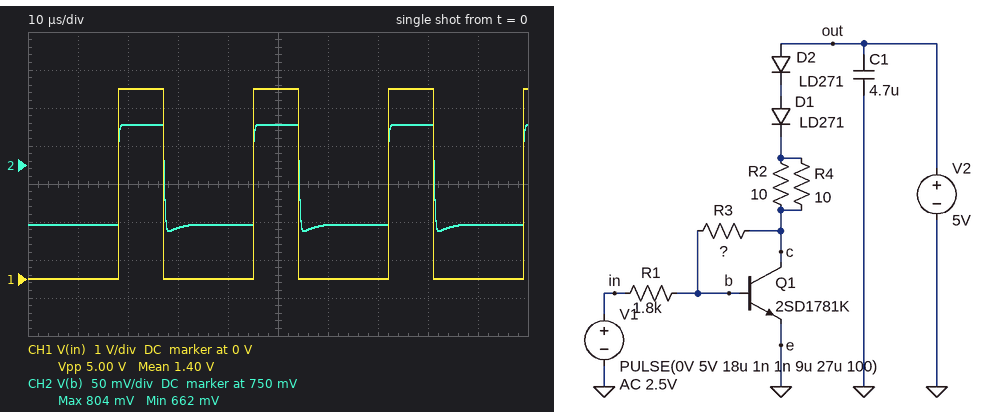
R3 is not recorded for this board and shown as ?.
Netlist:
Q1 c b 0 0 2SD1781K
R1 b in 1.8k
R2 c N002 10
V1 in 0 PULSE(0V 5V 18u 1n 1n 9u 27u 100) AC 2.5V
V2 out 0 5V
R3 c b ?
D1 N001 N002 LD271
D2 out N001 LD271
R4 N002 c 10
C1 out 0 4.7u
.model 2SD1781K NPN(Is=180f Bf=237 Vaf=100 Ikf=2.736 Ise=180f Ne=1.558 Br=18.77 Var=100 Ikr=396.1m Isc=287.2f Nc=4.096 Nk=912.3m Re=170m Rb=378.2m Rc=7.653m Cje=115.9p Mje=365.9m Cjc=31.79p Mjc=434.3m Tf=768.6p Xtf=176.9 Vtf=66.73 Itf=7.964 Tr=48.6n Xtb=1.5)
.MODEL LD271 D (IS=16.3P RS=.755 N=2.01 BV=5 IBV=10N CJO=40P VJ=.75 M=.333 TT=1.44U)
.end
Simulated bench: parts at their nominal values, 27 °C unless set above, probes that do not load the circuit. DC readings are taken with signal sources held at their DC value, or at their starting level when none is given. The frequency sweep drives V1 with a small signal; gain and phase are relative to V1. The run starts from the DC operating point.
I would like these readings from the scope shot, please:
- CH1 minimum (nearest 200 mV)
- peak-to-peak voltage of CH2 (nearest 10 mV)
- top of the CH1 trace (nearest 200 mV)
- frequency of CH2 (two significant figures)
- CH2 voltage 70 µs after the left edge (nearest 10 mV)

0 V
140 mV
5.0 V
37 kHz
670 mV
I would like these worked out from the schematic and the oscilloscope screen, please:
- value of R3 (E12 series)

3.9 kΩ
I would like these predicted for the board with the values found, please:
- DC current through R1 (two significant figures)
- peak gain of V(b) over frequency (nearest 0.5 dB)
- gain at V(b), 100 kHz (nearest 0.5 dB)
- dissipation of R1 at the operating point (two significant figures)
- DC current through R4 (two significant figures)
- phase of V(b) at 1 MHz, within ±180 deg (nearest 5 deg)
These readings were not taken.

370 µA
-21.5 dB
-21.5 dB
250 µW
14 mA
-45 deg
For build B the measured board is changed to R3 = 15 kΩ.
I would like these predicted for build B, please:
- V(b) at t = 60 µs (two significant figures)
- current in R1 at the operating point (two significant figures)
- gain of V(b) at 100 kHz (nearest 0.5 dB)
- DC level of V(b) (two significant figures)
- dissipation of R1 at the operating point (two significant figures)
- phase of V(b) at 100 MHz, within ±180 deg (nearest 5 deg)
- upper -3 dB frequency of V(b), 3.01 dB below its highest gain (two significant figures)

310 mV
200 µA
-1.0 dB
350 mV
70 µW
-85 deg
610 kHz
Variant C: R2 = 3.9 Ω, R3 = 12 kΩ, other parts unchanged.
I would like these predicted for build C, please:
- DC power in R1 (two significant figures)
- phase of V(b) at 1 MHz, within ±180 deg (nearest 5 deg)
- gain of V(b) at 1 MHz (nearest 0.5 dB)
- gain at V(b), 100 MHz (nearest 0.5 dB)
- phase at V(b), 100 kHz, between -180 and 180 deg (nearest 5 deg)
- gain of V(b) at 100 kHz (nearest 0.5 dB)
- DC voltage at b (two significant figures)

100 µW
-60 deg
-7.0 dB
-46.0 dB
-10 deg
-1.5 dB
430 mV
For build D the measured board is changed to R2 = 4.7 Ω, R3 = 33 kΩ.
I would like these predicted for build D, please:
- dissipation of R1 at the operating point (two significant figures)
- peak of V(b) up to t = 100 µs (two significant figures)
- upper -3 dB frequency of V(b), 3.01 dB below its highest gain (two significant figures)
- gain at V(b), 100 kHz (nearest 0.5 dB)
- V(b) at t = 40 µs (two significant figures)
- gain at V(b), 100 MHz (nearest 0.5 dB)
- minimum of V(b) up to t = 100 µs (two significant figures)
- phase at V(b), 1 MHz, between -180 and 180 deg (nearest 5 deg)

17 µW
810 mV
650 kHz
-0.5 dB
170 mV
-44.0 dB
140 mV
-55 deg
